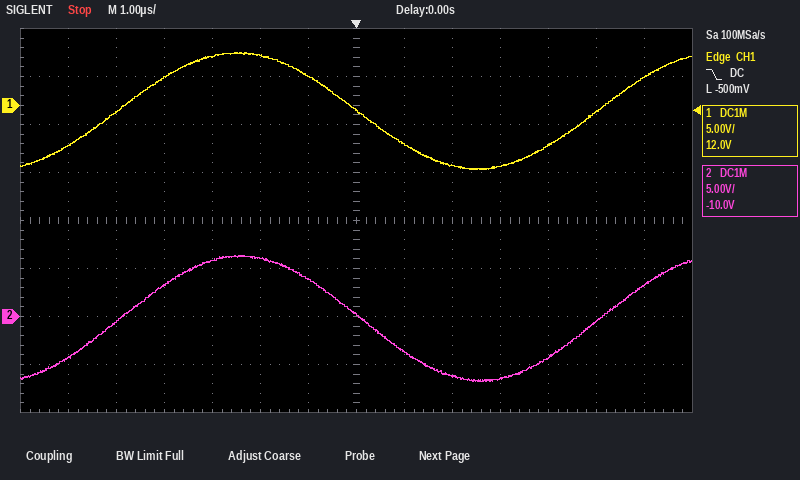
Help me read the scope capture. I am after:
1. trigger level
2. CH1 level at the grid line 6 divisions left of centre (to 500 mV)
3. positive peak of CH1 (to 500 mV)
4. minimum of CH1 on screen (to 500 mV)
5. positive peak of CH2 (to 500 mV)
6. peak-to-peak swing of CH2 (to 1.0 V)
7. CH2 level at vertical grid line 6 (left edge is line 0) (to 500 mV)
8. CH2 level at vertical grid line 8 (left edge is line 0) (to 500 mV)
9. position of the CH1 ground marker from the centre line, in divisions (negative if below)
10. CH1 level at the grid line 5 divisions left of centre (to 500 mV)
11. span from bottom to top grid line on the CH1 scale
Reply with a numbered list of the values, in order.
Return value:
1. -500 mV
2. -4.0 V
3. 5.5 V
4. -6.5 V
5. 6.5 V
6. 13.0 V
7. 4.0 V
8. -3.5 V
9. +2.4 div
10. -500 mV
11. 40 V
